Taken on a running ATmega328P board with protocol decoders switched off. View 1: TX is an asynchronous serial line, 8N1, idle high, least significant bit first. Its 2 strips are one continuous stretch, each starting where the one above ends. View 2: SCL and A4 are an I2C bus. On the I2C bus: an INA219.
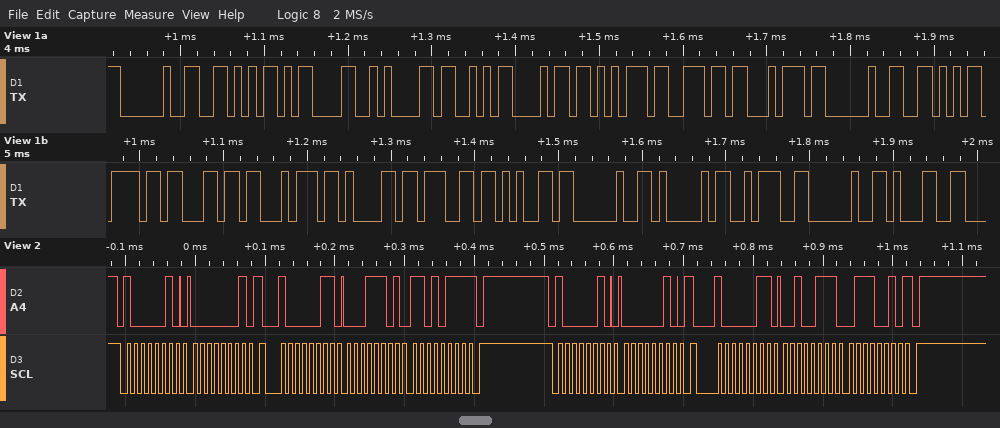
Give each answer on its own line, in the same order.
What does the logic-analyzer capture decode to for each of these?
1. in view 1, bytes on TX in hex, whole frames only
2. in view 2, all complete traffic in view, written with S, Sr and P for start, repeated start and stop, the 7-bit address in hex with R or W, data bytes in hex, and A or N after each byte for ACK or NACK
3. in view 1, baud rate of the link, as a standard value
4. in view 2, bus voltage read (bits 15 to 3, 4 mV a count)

20 56 0D 0A 53 68 75 6E 74 20 56 6F 6C 74 61 67 65 20 41 3A 20 31
S 41W A 01 A Sr 41R A 1D A D7 N P S 41W A 02 A Sr 41R A 27 A 72 N P
115200 baud
5.048 V
